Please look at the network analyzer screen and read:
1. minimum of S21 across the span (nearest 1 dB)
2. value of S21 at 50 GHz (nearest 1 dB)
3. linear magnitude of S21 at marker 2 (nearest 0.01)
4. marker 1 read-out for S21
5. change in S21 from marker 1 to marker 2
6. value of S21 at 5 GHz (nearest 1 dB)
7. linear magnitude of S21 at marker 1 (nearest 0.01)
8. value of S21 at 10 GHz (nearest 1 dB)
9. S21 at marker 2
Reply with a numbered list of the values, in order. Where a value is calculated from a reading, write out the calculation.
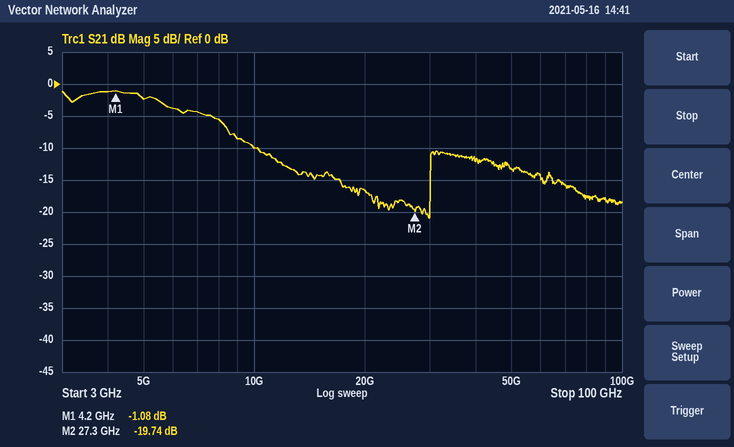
1. -21 dB
2. -13 dB
3. 10^(-19.74/20) ≈ 0.10
4. -1.08 dB
5. -19.74 − (-1.08) = -18.66 dB
6. -2 dB
7. 10^(-1.08/20) ≈ 0.88
8. -10 dB
9. -19.74 dB
